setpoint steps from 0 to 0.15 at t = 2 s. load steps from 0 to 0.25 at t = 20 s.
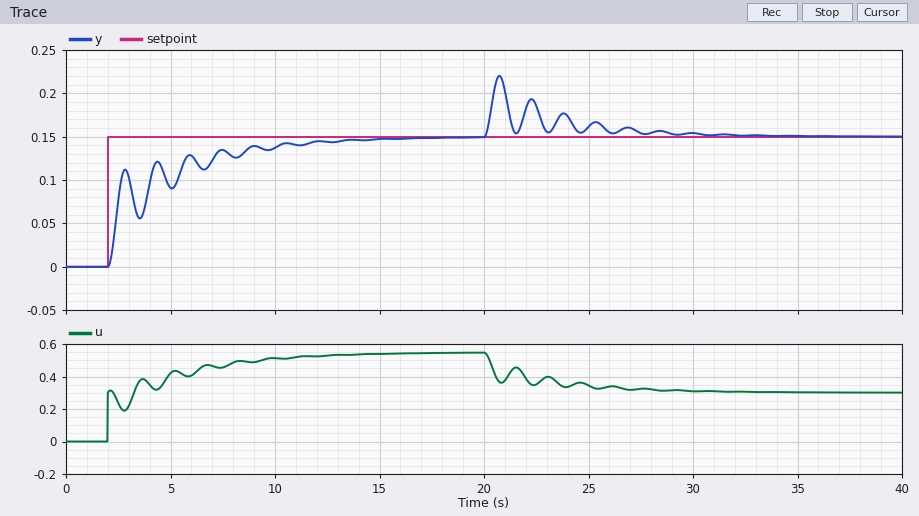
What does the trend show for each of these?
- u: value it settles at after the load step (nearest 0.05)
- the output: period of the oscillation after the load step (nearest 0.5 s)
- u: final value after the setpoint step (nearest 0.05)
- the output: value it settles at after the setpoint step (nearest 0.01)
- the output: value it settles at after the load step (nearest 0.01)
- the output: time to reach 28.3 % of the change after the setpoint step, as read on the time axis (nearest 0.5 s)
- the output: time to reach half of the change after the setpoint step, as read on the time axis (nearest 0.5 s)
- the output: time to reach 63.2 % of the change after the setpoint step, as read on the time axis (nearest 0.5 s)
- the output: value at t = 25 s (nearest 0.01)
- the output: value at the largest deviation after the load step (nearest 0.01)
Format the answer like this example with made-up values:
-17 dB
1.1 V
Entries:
0.30
1.5 s
0.55
0.15
0.15
2.5 s
2.5 s
2.5 s
0.16
0.22
